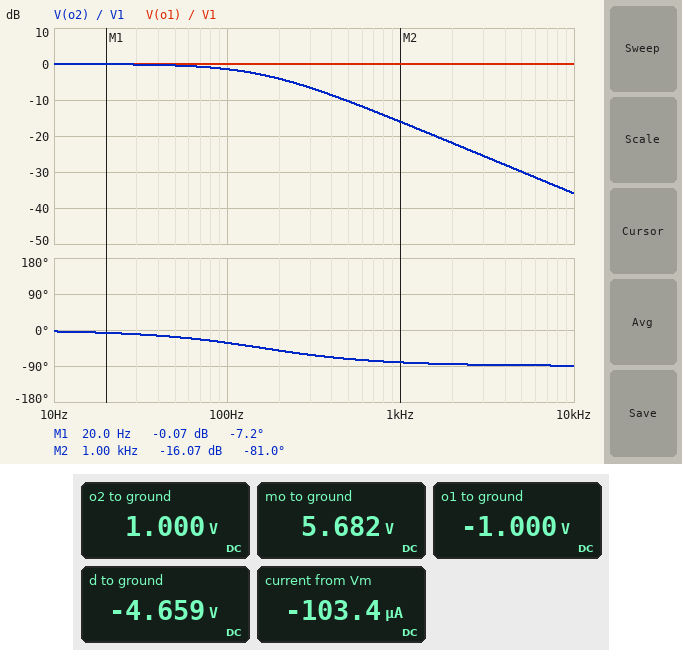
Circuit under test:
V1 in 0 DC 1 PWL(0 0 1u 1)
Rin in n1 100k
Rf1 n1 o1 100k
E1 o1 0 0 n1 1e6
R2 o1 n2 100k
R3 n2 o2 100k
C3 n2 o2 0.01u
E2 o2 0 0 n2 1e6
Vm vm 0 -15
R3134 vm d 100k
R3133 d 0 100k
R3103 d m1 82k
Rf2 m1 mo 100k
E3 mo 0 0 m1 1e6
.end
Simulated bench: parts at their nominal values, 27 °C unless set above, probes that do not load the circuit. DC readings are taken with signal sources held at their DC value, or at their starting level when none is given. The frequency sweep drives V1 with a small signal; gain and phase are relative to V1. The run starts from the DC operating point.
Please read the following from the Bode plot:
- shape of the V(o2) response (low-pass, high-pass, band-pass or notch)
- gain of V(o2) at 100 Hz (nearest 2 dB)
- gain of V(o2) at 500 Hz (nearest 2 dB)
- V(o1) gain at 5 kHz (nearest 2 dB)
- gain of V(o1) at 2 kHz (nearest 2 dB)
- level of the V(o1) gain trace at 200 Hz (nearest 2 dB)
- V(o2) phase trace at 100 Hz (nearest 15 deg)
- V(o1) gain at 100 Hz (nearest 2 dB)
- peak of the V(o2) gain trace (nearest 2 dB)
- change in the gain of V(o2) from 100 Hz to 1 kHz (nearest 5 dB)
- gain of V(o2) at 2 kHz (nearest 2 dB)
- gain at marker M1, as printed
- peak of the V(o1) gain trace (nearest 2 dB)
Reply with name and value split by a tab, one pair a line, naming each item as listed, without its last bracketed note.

shape of the V(o2) response	low-pass
gain of V(o2) at 100 Hz	-2 dB
gain of V(o2) at 500 Hz	-10 dB
V(o1) gain at 5 kHz	0 dB
gain of V(o1) at 2 kHz	0 dB
level of the V(o1) gain trace at 200 Hz	0 dB
V(o2) phase trace at 100 Hz	-30 deg
V(o1) gain at 100 Hz	0 dB
peak of the V(o2) gain trace	0 dB
change in the gain of V(o2) from 100 Hz to 1 kHz	-15 dB
gain of V(o2) at 2 kHz	-22 dB
gain at marker M1, as printed	-0.07 dB
peak of the V(o1) gain trace	0 dB
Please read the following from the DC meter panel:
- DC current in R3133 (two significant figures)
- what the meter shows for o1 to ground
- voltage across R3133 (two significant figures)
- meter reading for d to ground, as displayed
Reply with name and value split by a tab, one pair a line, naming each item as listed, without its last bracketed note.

DC current in R3133	47 µA
what the meter shows for o1 to ground	-1.000 V
voltage across R3133	4.7 V
meter reading for d to ground, as displayed	-4.659 V
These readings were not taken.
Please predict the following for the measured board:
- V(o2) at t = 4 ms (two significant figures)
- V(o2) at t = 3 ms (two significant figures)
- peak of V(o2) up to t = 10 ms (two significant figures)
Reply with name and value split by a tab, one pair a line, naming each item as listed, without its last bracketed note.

V(o2) at t = 4 ms	980 mV
V(o2) at t = 3 ms	950 mV
peak of V(o2) up to t = 10 ms	1.0 V
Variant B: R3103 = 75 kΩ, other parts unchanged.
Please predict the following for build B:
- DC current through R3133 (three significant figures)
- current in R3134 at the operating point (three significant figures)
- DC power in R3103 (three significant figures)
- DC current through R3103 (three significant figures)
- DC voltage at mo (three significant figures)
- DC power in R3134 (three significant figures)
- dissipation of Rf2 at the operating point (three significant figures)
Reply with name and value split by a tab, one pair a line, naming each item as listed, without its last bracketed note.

DC current through R3133	45.0 µA
current in R3134 at the operating point	105 µA
DC power in R3103	270 µW
DC current through R3103	60.0 µA
DC voltage at mo	6.00 V
DC power in R3134	1.10 mW
dissipation of Rf2 at the operating point	360 µW
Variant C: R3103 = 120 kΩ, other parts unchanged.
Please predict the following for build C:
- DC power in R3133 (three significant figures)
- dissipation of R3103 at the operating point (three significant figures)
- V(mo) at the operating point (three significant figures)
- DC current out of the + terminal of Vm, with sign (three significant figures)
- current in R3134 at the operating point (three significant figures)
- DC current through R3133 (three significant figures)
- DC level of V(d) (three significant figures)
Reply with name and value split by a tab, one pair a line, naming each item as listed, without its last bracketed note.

DC power in R3133	280 µW
dissipation of R3103 at the operating point	234 µW
V(mo) at the operating point	4.41 V
DC current out of the + terminal of Vm, with sign	-97.1 µA
current in R3134 at the operating point	97.1 µA
DC current through R3133	52.9 µA
DC level of V(d)	-5.29 V
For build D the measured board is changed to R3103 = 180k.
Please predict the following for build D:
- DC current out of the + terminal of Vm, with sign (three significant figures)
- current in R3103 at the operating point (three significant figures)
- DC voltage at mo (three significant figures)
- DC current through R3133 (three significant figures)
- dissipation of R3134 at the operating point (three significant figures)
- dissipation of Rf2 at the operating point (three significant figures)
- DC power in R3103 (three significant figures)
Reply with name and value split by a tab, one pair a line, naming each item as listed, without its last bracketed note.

DC current out of the + terminal of Vm, with sign	-91.3 µA
current in R3103 at the operating point	32.6 µA
DC voltage at mo	3.26 V
DC current through R3133	58.7 µA
dissipation of R3134 at the operating point	834 µW
dissipation of Rf2 at the operating point	106 µW
DC power in R3103	191 µW
